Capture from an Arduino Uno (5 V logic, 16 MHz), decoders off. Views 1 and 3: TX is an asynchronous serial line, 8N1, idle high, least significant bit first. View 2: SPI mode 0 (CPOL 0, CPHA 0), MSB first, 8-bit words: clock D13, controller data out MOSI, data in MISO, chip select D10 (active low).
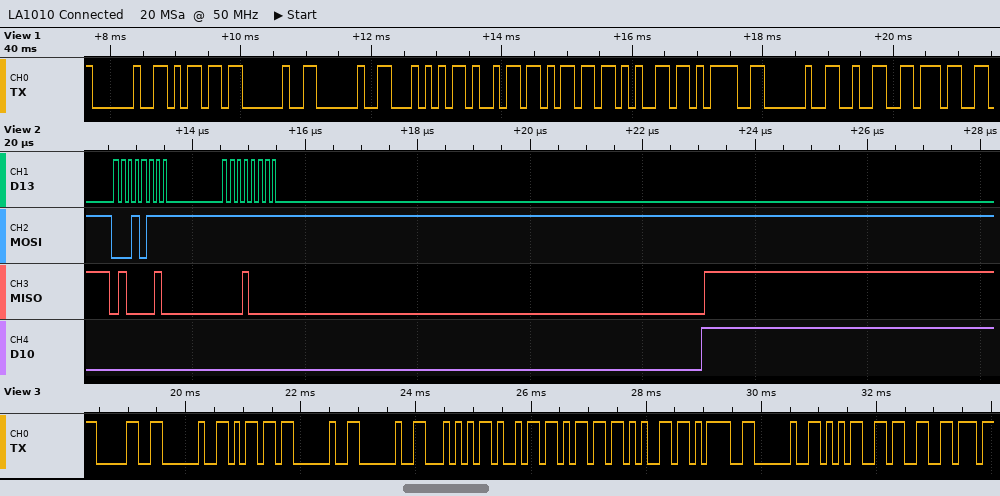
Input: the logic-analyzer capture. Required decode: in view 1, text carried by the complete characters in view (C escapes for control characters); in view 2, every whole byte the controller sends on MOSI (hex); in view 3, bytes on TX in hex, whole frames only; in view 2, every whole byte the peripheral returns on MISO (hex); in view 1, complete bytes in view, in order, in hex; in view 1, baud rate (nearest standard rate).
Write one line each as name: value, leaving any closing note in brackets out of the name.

in view 1, text carried by the complete characters in view: " m  Time= 27"
in view 2, every whole byte the controller sends on MOSI: 17 FF
in view 3, bytes on TX in hex, whole frames only: 30 20 6D 20 20 54 69 6D 65 3D 20 35 33
in view 2, every whole byte the peripheral returns on MISO: 42 10
in view 1, complete bytes in view, in order, in hex: 20 6D 20 20 54 69 6D 65 3D 20 32 37
in view 1, baud rate: 9600 baud
